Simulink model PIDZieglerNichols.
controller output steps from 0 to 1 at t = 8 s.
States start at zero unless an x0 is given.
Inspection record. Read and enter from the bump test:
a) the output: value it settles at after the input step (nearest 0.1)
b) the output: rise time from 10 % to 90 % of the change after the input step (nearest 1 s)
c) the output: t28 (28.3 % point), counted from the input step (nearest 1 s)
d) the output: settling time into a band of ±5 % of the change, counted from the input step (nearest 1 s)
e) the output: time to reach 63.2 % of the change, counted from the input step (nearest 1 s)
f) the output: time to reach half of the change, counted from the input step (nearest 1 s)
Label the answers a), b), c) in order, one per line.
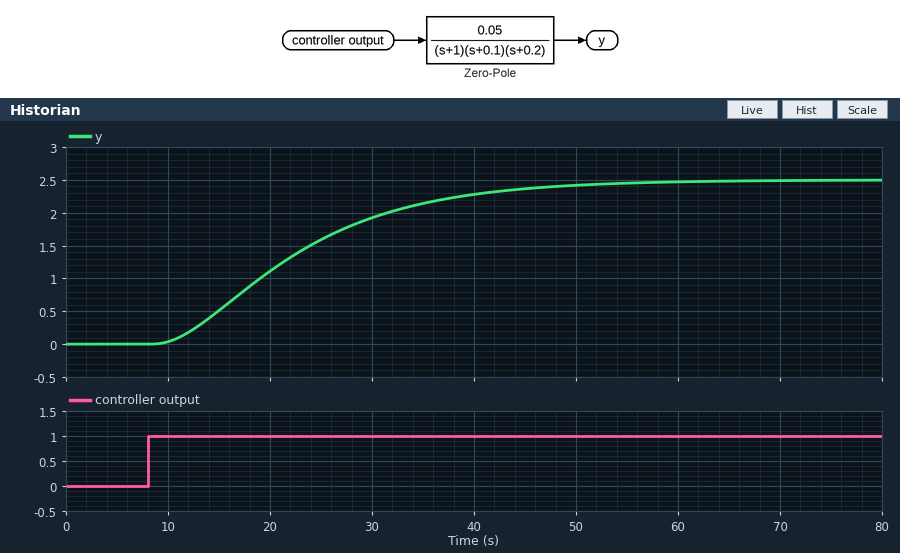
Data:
a) 2.5
b) 26 s
c) 9 s
d) 38 s
e) 17 s
f) 13 s
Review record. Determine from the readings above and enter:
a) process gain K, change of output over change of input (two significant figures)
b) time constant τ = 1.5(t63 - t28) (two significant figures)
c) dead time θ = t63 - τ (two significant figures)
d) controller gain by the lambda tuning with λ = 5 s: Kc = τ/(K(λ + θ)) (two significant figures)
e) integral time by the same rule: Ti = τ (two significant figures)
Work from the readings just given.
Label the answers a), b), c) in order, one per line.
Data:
a) 2.5
b) 12 s
c) 5.0 s
d) 0.48
e) 12 s
